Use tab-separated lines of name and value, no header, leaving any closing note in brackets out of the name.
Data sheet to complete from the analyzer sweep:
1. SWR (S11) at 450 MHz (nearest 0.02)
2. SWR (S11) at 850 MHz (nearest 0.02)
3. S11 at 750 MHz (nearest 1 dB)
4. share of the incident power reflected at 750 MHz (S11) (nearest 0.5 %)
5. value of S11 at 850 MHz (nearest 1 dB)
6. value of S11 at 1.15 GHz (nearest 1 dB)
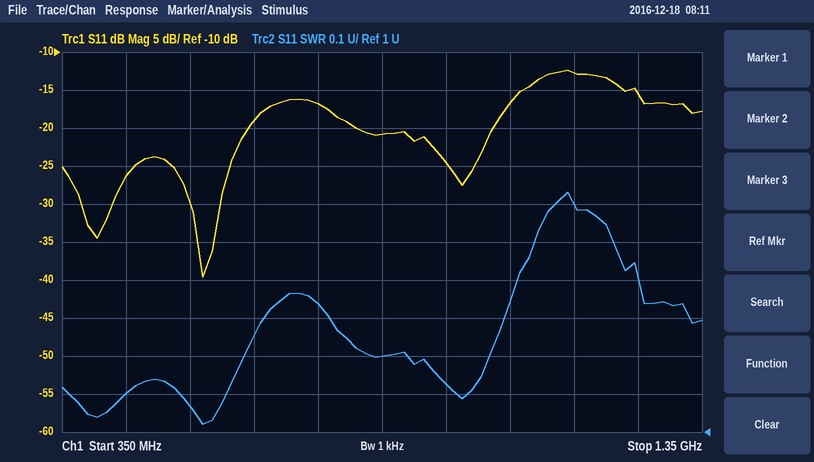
SWR (S11) at 450 MHz	1.10
SWR (S11) at 850 MHz	1.20
S11 at 750 MHz	-17 dB
share of the incident power reflected at 750 MHz (S11)	2.0 %
value of S11 at 850 MHz	-21 dB
value of S11 at 1.15 GHz	-13 dB
